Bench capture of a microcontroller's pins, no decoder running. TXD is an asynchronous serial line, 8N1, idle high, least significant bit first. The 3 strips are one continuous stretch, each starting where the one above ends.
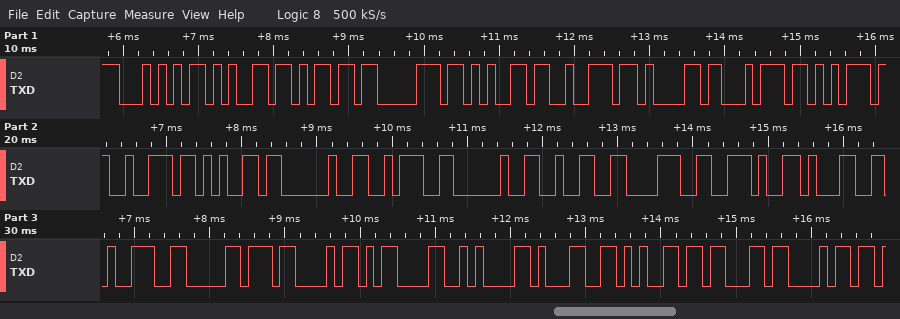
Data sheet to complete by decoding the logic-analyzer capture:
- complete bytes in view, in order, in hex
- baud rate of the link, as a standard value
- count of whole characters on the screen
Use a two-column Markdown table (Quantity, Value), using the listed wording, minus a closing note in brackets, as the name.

| Quantity | Value |
|---|---|
| complete bytes in view, in order, in hex | 54 65 6D 70 65 72 61 74 75 72 65 20 3A 20 32 38 2E 31 39 B0 43 0D 0A 31 65 63 68 |
| baud rate of the link, as a standard value | 9600 baud |
| count of whole characters on the screen | 27 |
